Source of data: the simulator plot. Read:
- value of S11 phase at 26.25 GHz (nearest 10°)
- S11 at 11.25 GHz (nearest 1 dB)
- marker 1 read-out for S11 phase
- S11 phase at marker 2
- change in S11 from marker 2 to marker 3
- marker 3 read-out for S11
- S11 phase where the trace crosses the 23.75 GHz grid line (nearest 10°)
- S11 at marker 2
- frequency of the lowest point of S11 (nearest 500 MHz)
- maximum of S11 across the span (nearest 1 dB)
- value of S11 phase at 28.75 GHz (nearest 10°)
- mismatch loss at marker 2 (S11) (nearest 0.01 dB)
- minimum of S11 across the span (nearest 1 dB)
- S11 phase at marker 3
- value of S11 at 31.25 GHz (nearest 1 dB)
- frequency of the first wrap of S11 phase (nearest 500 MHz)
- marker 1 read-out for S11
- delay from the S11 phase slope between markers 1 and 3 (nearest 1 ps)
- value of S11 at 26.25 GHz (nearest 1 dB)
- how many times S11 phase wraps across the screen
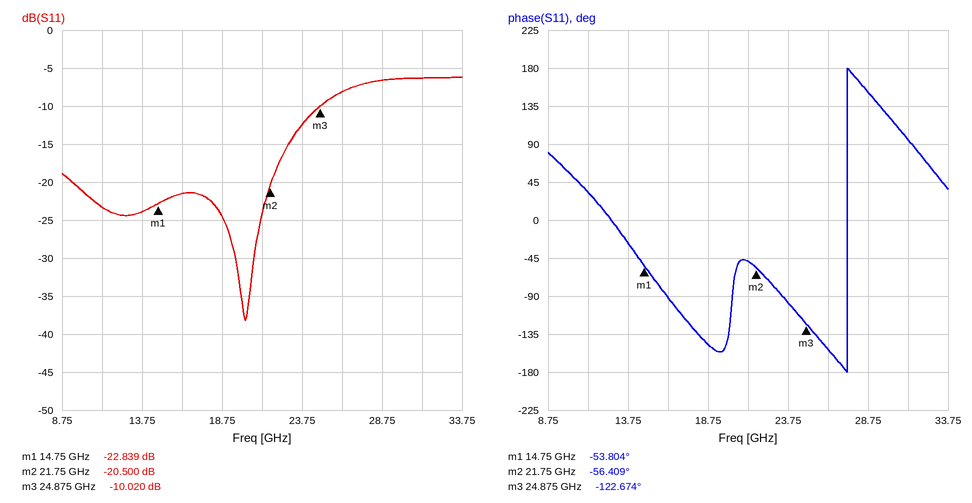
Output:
-150°
-23 dB
-53.804°
-56.409°
10.480 dB
-10.020 dB
-100°
-20.500 dB
20.0 GHz
-6 dB
150°
0.04 dB
-38 dB
-122.674°
-6 dB
27.5 GHz
-22.839 dB
19 ps
-8 dB
1
